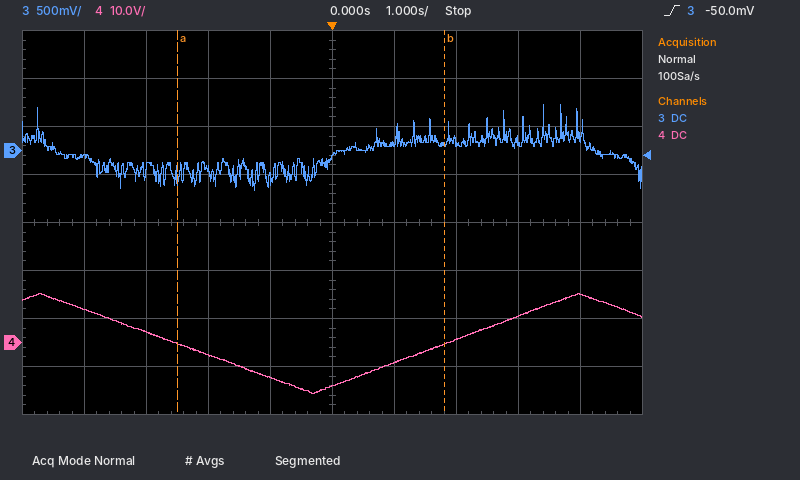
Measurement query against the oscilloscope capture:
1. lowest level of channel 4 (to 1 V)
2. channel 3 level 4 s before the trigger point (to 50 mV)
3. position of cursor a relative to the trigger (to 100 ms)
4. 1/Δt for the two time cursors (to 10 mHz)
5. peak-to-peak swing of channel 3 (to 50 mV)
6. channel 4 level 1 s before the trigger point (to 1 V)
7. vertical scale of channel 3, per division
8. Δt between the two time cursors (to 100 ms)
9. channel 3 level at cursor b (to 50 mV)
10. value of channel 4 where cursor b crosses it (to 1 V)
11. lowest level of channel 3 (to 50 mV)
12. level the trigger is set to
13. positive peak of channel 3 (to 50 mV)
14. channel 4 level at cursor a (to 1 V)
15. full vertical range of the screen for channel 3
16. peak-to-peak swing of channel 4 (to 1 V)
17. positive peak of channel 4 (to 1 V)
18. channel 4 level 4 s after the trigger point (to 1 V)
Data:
-11 V
-50 mV
-2.5 s
230 mHz
900 mV
-7 V
500 mV
4.3 s
100 mV
0 V
-400 mV
-50.0 mV
500 mV
0 V
4 V
21 V
10 V
10 V
